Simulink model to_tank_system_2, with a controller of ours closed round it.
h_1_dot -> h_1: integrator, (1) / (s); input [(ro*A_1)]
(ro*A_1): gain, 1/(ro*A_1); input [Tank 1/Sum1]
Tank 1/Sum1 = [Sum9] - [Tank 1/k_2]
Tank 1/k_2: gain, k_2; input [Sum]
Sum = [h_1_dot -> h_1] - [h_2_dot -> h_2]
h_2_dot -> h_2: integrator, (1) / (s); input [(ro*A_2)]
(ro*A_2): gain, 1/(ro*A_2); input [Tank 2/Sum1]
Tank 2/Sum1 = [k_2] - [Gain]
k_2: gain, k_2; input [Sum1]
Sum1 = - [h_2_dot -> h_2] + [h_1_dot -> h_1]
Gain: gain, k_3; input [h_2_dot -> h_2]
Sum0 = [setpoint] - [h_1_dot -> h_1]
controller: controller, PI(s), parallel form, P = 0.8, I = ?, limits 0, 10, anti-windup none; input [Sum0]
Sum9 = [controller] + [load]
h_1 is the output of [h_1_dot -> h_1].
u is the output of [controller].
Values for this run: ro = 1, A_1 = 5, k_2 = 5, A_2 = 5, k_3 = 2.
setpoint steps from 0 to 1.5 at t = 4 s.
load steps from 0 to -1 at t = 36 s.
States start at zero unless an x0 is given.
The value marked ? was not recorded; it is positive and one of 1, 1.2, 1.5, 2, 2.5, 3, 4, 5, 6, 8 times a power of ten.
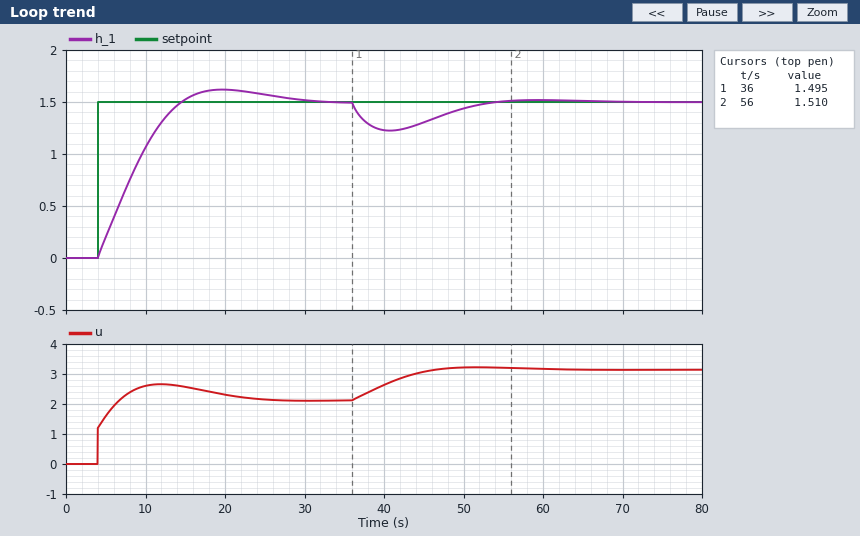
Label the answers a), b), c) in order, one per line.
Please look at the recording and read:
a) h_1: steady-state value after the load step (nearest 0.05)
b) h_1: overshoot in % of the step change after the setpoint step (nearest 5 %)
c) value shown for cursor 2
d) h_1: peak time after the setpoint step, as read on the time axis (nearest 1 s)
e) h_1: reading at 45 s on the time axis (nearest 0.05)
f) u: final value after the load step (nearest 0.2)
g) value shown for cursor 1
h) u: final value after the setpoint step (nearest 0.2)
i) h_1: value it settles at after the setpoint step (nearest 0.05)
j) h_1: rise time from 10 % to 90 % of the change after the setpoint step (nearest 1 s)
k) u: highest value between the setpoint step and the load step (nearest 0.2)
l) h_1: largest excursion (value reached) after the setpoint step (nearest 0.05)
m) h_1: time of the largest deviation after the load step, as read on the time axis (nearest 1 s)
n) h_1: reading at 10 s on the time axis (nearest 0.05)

a) 1.50
b) 10 %
c) 1.510
d) 20 s
e) 1.30
f) 3.2
g) 1.495
h) 2.2
i) 1.50
j) 8 s
k) 2.6
l) 1.60
m) 41 s
n) 1.05
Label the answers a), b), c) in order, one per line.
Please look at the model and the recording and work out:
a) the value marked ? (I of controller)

a) 0.4
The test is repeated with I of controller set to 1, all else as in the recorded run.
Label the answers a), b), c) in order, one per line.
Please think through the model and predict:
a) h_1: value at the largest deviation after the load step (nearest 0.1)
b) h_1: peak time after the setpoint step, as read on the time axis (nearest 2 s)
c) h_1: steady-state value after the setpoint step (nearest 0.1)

a) 1.3
b) 12 s
c) 1.5
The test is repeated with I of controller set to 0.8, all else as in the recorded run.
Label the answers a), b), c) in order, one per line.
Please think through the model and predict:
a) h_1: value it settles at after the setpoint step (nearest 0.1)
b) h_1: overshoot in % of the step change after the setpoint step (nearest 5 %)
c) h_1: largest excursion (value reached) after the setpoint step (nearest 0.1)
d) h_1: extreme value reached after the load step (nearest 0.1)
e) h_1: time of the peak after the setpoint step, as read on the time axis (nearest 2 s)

a) 1.5
b) 20 %
c) 1.8
d) 1.3
e) 14 s
